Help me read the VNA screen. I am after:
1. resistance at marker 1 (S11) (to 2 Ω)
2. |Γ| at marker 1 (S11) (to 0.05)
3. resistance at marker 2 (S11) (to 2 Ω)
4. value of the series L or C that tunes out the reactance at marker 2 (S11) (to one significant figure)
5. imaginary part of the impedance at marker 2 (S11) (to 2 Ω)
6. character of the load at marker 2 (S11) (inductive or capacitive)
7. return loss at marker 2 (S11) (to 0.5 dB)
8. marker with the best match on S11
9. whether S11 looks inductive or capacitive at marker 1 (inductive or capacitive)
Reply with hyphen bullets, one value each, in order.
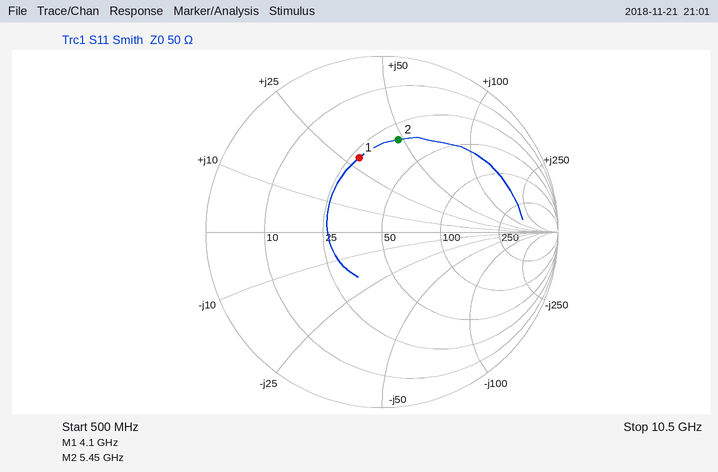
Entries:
- 28 Ω
- 0.45
- 32 Ω
- 600 fF
- +48 Ω
- inductive
- 5.5 dB
- marker 1
- inductive
